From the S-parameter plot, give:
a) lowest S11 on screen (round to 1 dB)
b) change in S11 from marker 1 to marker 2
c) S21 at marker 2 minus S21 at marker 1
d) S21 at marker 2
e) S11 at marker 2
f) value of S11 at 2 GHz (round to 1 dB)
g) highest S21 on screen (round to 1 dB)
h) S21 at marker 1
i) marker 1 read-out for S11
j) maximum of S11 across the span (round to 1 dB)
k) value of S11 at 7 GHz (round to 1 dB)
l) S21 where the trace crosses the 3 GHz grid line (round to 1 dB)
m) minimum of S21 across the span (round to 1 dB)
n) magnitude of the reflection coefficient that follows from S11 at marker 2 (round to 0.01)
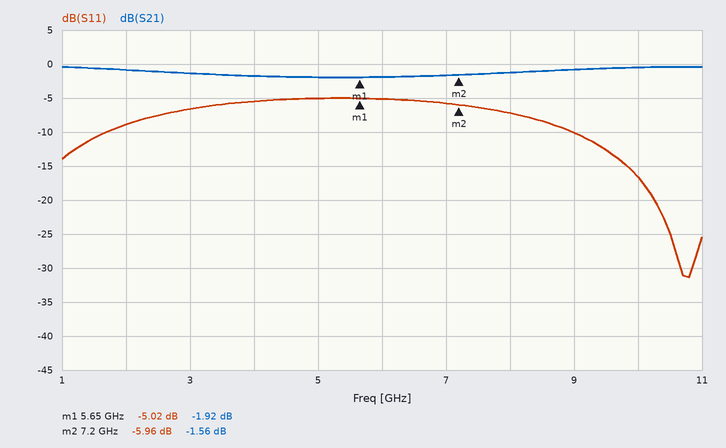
-31 dB
-0.94 dB
0.36 dB
-1.56 dB
-5.96 dB
-9 dB
0 dB
-1.92 dB
-5.02 dB
-5 dB
-6 dB
-1 dB
-2 dB
0.50
